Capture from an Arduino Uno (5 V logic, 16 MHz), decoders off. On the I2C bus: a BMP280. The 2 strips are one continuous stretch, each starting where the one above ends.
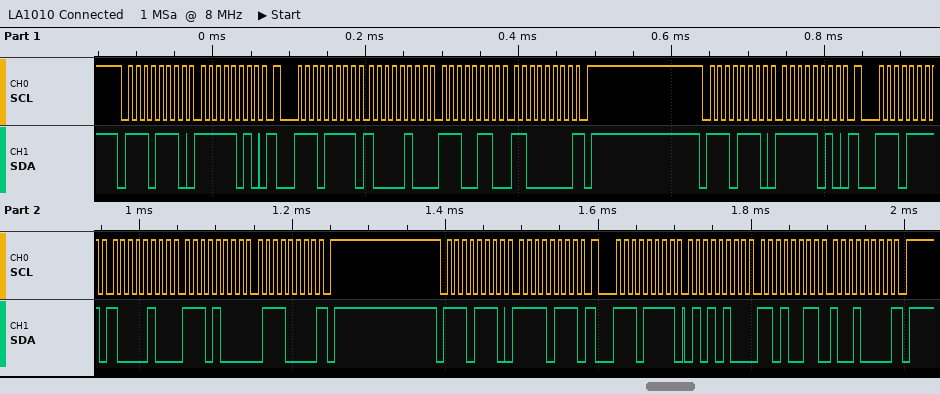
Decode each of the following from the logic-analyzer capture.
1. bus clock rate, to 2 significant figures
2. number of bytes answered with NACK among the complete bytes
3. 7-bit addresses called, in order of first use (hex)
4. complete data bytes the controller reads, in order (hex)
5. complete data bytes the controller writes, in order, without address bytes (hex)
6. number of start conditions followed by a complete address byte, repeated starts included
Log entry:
100 kHz
3
0x77
84 E6 C0 84 E8 70 54 D3 90
FA FA F7
6
